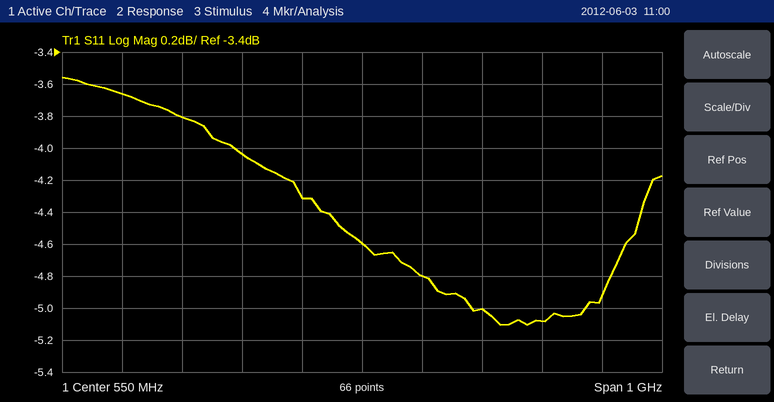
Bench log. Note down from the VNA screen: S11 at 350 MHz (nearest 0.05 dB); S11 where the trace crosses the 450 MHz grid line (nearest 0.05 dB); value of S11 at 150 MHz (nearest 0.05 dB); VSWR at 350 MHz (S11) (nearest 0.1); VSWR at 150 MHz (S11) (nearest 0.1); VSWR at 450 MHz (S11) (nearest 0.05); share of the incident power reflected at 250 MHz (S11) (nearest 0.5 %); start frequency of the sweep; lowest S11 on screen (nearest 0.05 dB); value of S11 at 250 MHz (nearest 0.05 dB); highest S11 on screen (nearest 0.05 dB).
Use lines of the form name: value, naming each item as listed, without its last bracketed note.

S11 at 350 MHz: -4.05 dB
S11 where the trace crosses the 450 MHz grid line: -4.30 dB
value of S11 at 150 MHz: -3.65 dB
VSWR at 350 MHz (S11): 4.4
VSWR at 150 MHz (S11): 4.8
VSWR at 450 MHz (S11): 4.10
share of the incident power reflected at 250 MHz (S11): 41.5 %
start frequency of the sweep: 50 MHz
lowest S11 on screen: -5.10 dB
value of S11 at 250 MHz: -3.80 dB
highest S11 on screen: -3.55 dB
